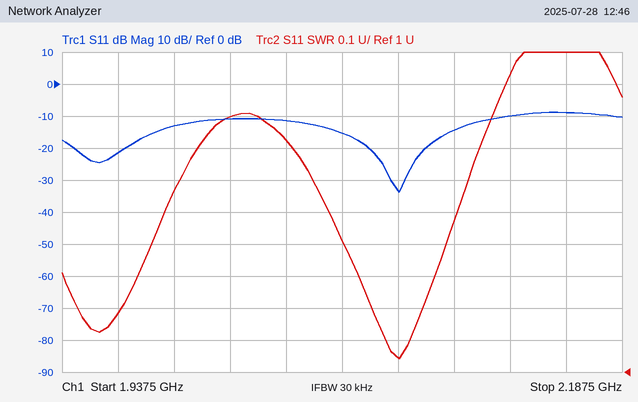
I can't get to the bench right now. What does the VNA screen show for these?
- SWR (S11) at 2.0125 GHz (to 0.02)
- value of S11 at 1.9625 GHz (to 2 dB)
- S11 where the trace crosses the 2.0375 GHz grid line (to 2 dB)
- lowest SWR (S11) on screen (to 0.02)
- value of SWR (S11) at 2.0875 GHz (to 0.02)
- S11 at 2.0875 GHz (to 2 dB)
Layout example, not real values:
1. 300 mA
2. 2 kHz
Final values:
1. 1.80
2. -22 dB
3. -12 dB
4. 1.04
5. 1.04
6. -34 dB
